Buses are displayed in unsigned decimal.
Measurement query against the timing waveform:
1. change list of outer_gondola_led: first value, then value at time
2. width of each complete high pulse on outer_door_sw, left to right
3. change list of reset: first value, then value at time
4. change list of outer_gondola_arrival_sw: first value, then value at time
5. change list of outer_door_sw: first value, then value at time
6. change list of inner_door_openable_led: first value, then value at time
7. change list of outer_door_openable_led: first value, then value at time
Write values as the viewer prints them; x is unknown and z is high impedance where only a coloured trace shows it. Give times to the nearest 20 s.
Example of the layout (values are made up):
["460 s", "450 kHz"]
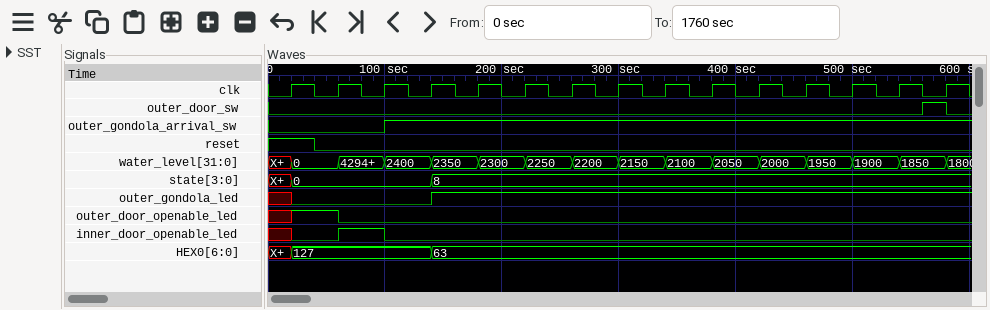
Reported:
["x, 0 at 20 s, 1 at 140 s", "20 s", "1, 0 at 40 s", "0, 1 at 100 s", "0, 1 at 560 s, 0 at 580 s", "x, 0 at 20 s, 1 at 60 s, 0 at 100 s", "x, 1 at 20 s, 0 at 60 s"]
